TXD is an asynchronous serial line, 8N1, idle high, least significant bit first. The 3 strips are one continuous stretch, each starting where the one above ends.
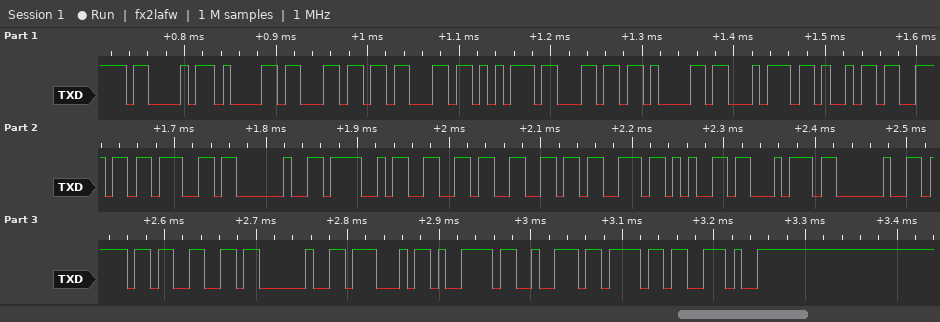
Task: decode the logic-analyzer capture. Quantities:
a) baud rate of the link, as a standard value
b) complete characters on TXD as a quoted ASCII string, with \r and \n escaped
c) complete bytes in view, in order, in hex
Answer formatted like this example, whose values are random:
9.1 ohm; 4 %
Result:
115200 baud; "Calculating Offset of Gyro."; 43 61 6C 63 75 6C 61 74 69 6E 67 20 4F 66 66 73 65 74 20 6F 66 20 47 79 72 6F 2E
